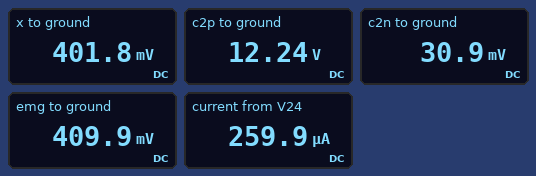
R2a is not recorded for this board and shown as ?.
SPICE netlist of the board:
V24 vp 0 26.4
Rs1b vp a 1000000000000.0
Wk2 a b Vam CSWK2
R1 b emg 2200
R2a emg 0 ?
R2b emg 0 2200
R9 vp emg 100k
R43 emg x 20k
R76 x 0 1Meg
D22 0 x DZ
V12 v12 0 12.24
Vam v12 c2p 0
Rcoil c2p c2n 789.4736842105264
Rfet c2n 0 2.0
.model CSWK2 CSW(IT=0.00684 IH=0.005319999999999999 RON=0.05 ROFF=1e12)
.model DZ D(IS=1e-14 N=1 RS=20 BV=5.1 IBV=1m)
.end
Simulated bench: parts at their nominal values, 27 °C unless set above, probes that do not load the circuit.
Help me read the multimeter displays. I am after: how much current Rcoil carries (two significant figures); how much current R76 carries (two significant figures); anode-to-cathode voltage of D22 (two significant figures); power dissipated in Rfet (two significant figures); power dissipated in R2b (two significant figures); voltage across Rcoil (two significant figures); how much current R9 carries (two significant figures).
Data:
15 mA
400 nA
-400 mV
480 µW
76 µW
12 V
260 µA
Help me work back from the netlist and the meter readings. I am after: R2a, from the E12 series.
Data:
5.6 kΩ
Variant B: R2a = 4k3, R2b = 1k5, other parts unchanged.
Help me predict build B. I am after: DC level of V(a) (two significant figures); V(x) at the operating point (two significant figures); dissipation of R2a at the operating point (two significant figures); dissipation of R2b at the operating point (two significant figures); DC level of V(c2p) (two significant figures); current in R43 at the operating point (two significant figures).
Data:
290 mV
280 mV
20 µW
56 µW
12 V
280 nA
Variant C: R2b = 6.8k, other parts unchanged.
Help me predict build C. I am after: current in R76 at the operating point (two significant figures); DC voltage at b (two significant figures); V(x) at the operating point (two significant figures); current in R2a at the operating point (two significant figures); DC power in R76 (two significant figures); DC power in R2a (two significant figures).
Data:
770 nA
780 mV
770 mV
140 µA
590 nW
110 µW
